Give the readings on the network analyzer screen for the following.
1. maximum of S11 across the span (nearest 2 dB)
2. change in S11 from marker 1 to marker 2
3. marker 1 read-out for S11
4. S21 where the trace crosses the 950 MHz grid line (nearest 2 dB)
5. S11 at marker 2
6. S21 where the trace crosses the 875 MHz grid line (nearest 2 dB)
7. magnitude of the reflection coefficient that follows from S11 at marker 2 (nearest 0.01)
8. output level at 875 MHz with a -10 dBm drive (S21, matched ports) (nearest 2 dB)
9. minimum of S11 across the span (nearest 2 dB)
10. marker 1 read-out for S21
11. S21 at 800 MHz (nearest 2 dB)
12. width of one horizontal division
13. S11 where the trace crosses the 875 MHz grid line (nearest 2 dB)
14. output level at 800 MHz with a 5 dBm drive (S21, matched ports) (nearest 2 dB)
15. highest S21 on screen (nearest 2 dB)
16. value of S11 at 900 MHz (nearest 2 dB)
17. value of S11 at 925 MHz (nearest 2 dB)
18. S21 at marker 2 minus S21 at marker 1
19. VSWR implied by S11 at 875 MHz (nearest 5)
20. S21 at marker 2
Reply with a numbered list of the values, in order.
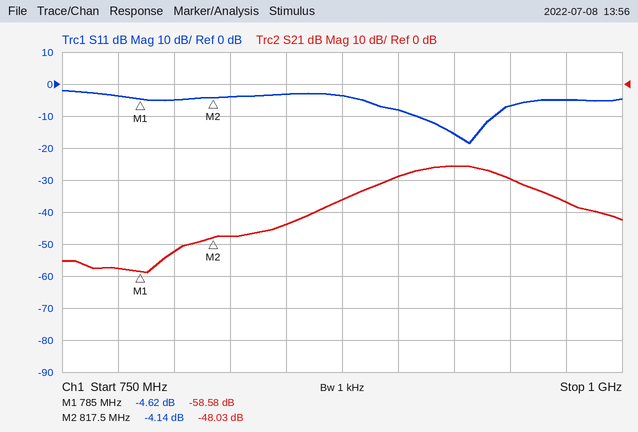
1. -2 dB
2. 0.48 dB
3. -4.62 dB
4. -30 dB
5. -4.14 dB
6. -36 dB
7. 0.62
8. -46 dBm
9. -18 dB
10. -58.58 dB
11. -52 dB
12. 25 MHz
13. -4 dB
14. -48 dBm
15. -26 dB
16. -8 dB
17. -16 dB
18. 10.55 dB
19. 5
20. -48.03 dB
